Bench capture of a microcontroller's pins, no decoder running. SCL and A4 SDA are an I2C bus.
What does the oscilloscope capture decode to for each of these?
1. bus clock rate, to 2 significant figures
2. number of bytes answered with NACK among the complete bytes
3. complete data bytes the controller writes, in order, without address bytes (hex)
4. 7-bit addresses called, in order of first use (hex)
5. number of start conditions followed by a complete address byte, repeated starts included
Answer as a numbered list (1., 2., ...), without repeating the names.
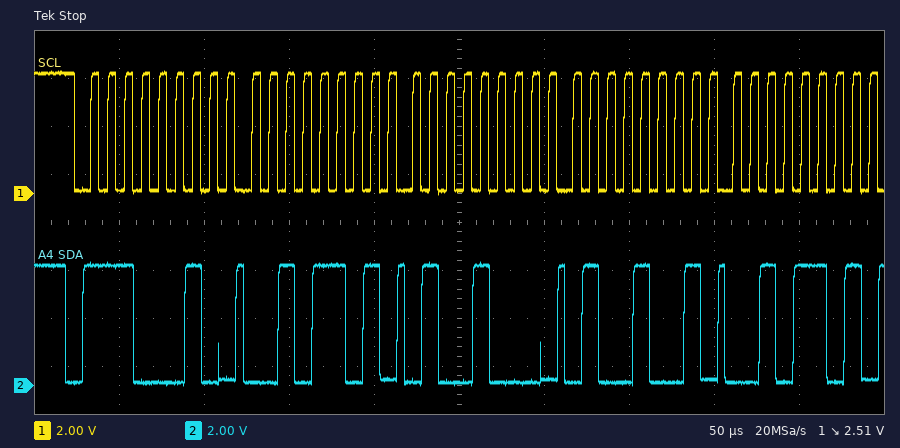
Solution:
1. 100 kHz
2. 0
3. 2D 48 49 2D
4. 0x71
5. 1
